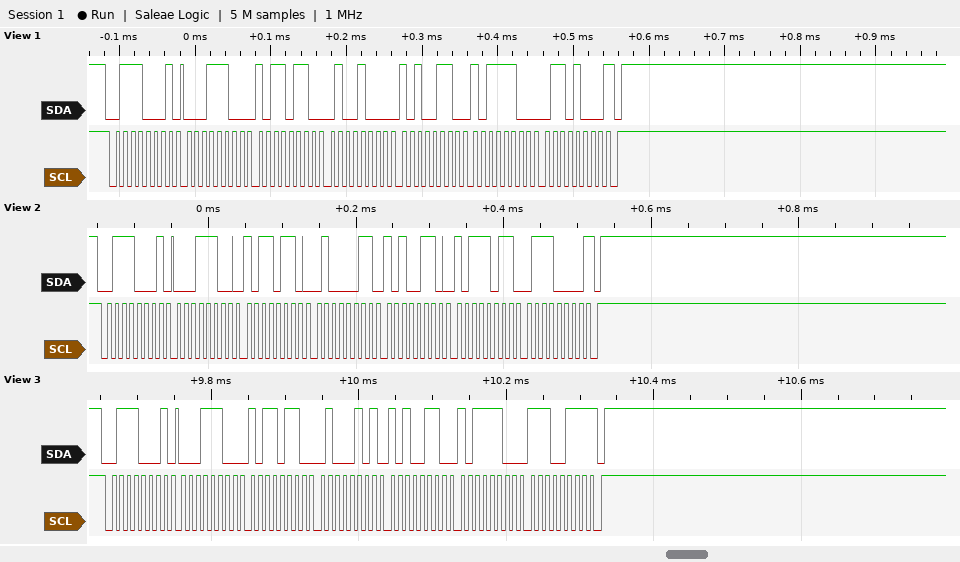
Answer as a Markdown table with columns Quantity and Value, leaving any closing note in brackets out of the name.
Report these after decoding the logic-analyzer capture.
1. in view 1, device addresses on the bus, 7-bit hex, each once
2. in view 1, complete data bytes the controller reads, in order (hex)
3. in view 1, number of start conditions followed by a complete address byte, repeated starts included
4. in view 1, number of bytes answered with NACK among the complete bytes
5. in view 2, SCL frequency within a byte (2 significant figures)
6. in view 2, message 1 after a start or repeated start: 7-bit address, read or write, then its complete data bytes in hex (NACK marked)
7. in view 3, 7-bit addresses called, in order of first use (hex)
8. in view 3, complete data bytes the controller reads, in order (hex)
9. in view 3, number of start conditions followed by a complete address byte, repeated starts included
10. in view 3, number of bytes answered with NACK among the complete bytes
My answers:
| Quantity | Value |
|---|---|
| in view 1, device addresses on the bus, 7-bit hex, each once | 0x38 |
| in view 1, complete data bytes the controller reads, in order | 1C B6 48 A6 BC 68 |
| in view 1, number of start conditions followed by a complete address byte, repeated starts included | 1 |
| in view 1, number of bytes answered with NACK among the complete bytes | 1 |
| in view 2, SCL frequency within a byte | 100 kHz |
| in view 2, message 1 after a start or repeated start: 7-bit address, read or write, then its complete data bytes in hex | 0x38 read: 1C B6 43 A6 BB 70 NACK |
| in view 3, 7-bit addresses called, in order of first use | 0x38 |
| in view 3, complete data bytes the controller reads, in order | 1C B6 45 A6 BC E7 |
| in view 3, number of start conditions followed by a complete address byte, repeated starts included | 1 |
| in view 3, number of bytes answered with NACK among the complete bytes | 1 |
